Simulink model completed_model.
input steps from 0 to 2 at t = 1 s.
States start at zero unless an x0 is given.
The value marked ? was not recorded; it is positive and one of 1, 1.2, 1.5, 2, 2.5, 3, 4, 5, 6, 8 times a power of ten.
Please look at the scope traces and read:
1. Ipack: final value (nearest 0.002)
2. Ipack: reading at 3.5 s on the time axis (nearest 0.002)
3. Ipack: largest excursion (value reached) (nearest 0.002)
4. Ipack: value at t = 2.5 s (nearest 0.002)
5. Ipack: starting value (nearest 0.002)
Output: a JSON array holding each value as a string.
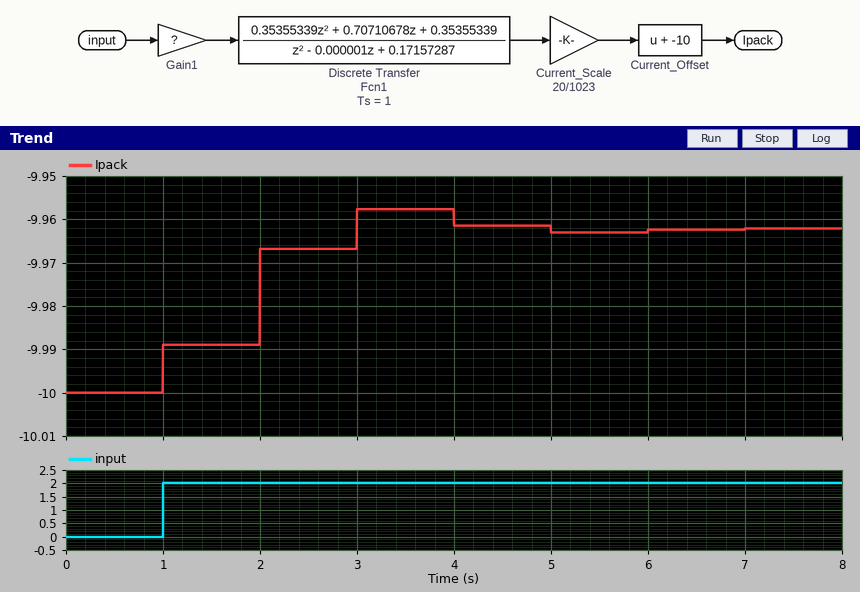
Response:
["-9.962", "-9.958", "-9.958", "-9.966", "-10.000"]
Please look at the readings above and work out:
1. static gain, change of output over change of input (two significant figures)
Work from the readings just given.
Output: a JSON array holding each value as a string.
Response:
["0.019"]
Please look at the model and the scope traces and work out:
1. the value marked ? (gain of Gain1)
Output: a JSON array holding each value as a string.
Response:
["0.8"]
